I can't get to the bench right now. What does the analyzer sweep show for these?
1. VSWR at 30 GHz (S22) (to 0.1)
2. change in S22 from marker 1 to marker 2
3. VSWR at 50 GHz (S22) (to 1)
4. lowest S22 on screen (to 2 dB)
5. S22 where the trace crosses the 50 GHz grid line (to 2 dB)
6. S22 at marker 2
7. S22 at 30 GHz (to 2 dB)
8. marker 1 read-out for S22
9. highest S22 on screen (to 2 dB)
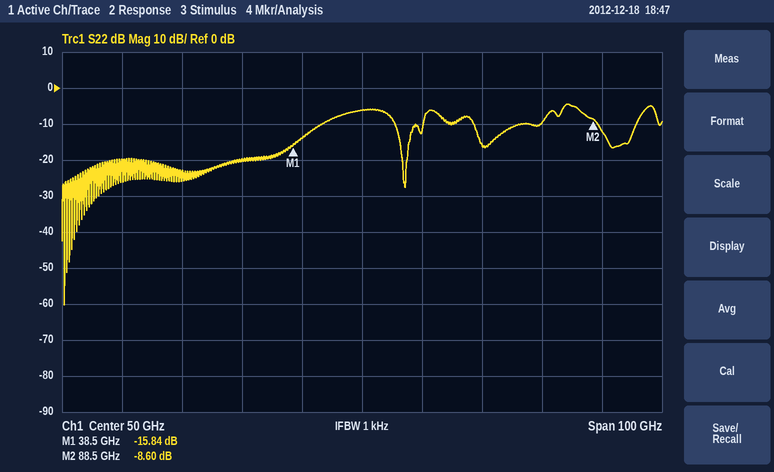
1.2
7.24 dB
3
-60 dB
-6 dB
-8.60 dB
-20 dB
-15.84 dB
-4 dB
